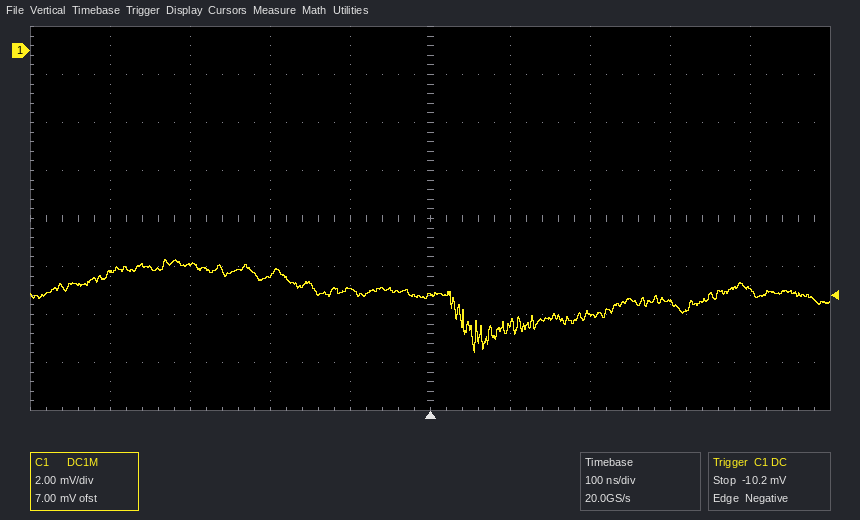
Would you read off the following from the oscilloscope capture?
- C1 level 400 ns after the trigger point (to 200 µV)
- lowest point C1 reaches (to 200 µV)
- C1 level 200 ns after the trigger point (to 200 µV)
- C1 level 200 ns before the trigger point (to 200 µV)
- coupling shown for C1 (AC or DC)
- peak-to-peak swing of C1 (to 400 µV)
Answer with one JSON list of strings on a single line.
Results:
["-10.0 mV", "-12.6 mV", "-11.0 mV", "-9.4 mV", "DC", "4.0 mV"]
